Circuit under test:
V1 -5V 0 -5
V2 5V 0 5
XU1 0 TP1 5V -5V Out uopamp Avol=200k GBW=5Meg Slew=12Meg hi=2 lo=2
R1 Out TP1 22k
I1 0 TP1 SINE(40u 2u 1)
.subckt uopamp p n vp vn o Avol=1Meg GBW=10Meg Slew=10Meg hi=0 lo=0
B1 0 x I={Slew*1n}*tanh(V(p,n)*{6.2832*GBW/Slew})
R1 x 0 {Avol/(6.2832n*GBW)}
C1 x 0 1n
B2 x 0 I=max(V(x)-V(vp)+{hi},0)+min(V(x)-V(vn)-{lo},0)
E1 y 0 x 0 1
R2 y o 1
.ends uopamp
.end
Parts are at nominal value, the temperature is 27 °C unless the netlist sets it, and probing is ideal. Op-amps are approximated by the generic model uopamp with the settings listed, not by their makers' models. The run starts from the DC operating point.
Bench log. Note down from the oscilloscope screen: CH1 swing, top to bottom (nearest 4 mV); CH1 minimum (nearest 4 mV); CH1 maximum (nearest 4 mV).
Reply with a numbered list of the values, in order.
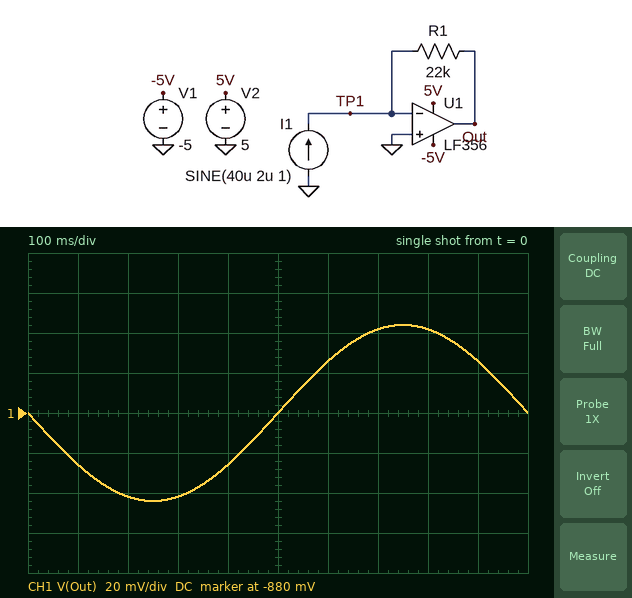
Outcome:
1. 88 mV
2. -924 mV
3. -836 mV
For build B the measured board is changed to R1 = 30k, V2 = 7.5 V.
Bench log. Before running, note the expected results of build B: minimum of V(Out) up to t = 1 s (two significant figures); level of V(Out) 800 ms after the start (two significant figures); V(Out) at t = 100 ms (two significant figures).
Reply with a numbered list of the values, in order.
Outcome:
1. -1.3 V
2. -1.1 V
3. -1.2 V
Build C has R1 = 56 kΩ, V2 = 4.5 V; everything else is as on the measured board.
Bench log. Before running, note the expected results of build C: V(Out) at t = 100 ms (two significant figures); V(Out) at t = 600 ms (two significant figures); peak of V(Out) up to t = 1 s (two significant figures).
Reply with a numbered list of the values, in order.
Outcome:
1. -2.3 V
2. -2.2 V
3. -2.1 V
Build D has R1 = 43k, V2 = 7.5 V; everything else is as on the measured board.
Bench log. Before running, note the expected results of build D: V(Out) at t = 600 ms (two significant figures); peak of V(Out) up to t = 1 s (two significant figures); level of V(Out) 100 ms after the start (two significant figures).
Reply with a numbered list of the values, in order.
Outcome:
1. -1.7 V
2. -1.6 V
3. -1.8 V
